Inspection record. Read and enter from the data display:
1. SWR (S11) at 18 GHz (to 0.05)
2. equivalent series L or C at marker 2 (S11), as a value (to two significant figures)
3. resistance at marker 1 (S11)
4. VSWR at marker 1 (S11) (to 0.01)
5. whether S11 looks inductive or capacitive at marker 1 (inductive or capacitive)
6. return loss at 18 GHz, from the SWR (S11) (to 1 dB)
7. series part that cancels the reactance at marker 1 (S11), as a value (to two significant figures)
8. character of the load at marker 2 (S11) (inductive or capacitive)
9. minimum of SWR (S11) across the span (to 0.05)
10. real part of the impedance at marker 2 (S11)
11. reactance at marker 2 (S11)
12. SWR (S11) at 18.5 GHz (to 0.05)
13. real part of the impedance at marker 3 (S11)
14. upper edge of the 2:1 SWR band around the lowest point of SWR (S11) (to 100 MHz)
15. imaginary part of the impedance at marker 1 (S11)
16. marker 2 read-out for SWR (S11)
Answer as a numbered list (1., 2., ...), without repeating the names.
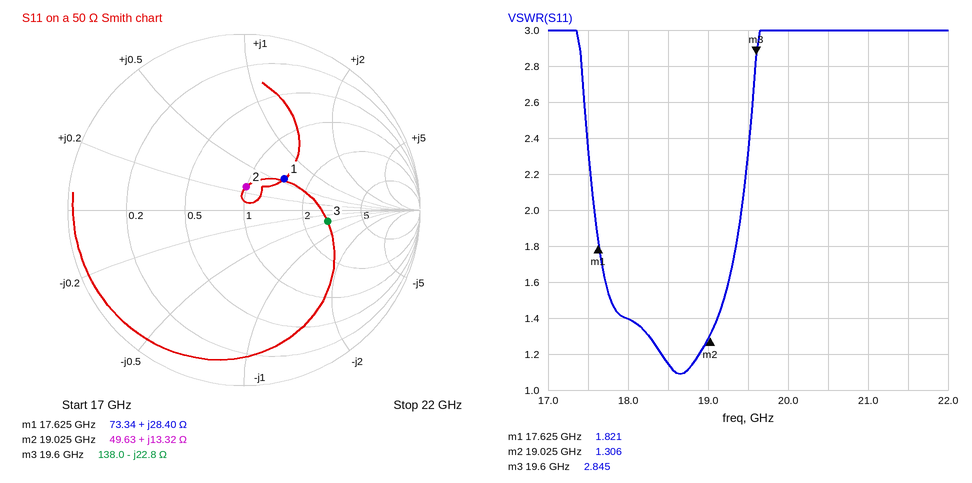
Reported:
1. 1.40
2. 110 pH
3. 73.34 Ω
4. 1.82
5. inductive
6. 16 dB
7. 320 fF
8. inductive
9. 1.10
10. 49.63 Ω
11. +13.32 Ω
12. 1.15
13. 138.0 Ω
14. 19.4 GHz
15. +28.40 Ω
16. 1.306
